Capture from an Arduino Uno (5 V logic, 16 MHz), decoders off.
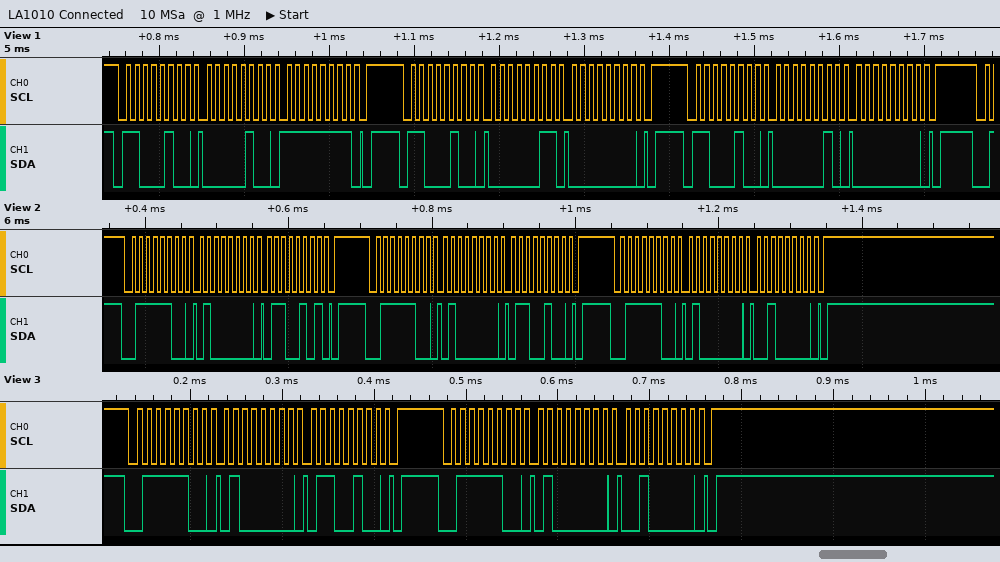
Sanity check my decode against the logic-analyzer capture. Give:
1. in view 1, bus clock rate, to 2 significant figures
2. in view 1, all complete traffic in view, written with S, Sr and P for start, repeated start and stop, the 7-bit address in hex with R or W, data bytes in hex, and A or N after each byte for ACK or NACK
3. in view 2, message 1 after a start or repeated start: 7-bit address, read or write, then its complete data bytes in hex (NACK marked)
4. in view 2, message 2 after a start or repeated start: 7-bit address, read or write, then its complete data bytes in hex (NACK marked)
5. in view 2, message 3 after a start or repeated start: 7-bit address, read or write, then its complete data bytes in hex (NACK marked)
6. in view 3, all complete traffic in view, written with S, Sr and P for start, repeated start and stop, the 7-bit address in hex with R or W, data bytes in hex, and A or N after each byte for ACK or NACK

100 kHz
S 62W A 04 A FF A P S 62W A 03 A 00 A P S 62W A 02 A 00 A P
0x3E write: 40 65
0x3E write: 40 64
0x3E write: 40 20
S 3EW A 40 A 64 A P S 3EW A 40 A 20 A P
